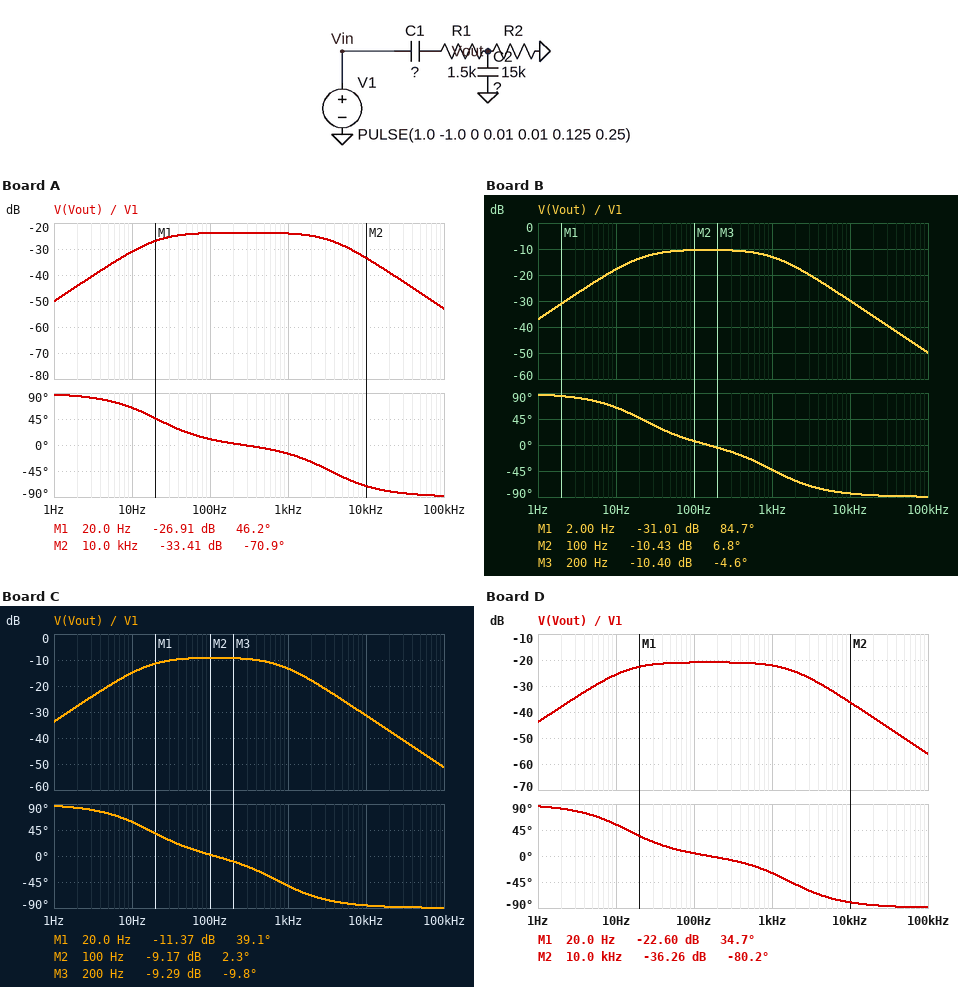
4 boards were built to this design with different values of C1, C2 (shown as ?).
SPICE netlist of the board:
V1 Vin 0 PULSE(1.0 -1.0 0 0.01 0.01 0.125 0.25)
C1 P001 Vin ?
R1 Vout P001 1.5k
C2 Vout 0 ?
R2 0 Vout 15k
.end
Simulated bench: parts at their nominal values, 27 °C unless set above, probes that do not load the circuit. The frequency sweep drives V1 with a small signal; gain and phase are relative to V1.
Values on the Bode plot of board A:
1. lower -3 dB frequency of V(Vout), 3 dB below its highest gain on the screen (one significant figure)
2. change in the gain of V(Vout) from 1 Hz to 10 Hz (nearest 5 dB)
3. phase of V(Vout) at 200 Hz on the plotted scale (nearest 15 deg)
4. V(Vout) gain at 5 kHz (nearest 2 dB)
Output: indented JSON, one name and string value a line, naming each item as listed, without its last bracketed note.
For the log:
{
  "lower -3 dB frequency of V(Vout), 3 dB below its highest gain on the screen": "20 Hz",
  "change in the gain of V(Vout) from 1 Hz to 10 Hz": "20 dB",
  "phase of V(Vout) at 200 Hz on the plotted scale": "0 deg",
  "V(Vout) gain at 5 kHz": "-28 dB"
}
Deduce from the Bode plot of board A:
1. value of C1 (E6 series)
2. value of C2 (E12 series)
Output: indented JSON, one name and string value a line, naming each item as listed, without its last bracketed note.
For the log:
{
  "value of C1": "33 nF",
  "value of C2": "470 nF"
}
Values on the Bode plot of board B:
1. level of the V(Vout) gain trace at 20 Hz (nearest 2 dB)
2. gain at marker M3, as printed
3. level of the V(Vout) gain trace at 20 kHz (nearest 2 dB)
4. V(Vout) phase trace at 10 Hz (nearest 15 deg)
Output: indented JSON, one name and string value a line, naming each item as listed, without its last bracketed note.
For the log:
{
  "level of the V(Vout) gain trace at 20 Hz": "-14 dB",
  "gain at marker M3, as printed": "-10.40 dB",
  "level of the V(Vout) gain trace at 20 kHz": "-36 dB",
  "V(Vout) phase trace at 10 Hz": "60 deg"
}
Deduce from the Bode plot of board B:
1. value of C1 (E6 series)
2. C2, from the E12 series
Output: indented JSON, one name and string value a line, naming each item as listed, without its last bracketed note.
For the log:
{
  "value of C1": "150 nF",
  "C2, from the E12 series": "330 nF"
}
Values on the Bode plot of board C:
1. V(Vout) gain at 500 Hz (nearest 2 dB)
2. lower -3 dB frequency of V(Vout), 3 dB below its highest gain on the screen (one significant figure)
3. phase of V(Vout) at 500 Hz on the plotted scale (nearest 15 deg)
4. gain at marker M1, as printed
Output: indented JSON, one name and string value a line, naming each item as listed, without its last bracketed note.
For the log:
{
  "V(Vout) gain at 500 Hz": "-10 dB",
  "lower -3 dB frequency of V(Vout), 3 dB below its highest gain on the screen": "20 Hz",
  "phase of V(Vout) at 500 Hz on the plotted scale": "-30 deg",
  "gain at marker M1, as printed": "-11.37 dB"
}
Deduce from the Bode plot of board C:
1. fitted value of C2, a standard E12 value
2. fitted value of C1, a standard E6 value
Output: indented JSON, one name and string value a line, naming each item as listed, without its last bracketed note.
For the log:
{
  "fitted value of C2, a standard E12 value": "390 nF",
  "fitted value of C1, a standard E6 value": "220 nF"
}
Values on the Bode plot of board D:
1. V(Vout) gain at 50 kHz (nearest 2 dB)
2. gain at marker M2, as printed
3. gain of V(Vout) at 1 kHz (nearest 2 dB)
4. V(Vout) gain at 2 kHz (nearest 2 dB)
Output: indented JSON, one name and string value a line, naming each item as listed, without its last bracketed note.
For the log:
{
  "V(Vout) gain at 50 kHz": "-50 dB",
  "gain at marker M2, as printed": "-36.26 dB",
  "gain of V(Vout) at 1 kHz": "-22 dB",
  "V(Vout) gain at 2 kHz": "-24 dB"
}
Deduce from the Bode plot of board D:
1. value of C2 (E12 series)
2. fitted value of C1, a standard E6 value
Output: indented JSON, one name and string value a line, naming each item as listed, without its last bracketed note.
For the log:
{
  "value of C2": "680 nF",
  "fitted value of C1, a standard E6 value": "68 nF"
}
